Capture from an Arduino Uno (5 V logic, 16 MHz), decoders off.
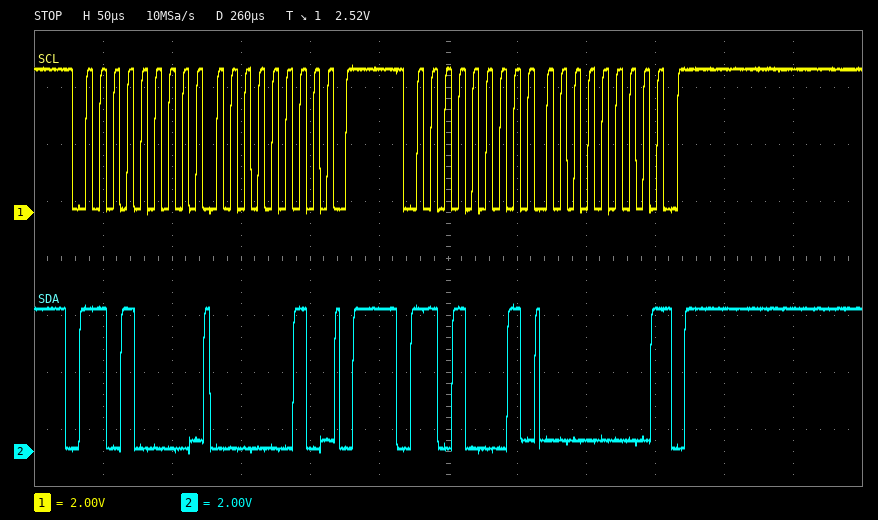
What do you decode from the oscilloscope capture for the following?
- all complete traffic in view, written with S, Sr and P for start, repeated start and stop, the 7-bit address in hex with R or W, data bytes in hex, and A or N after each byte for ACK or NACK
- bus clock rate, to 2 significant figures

S 68W A 02 A P S 68R A 00 N P
100 kHz
